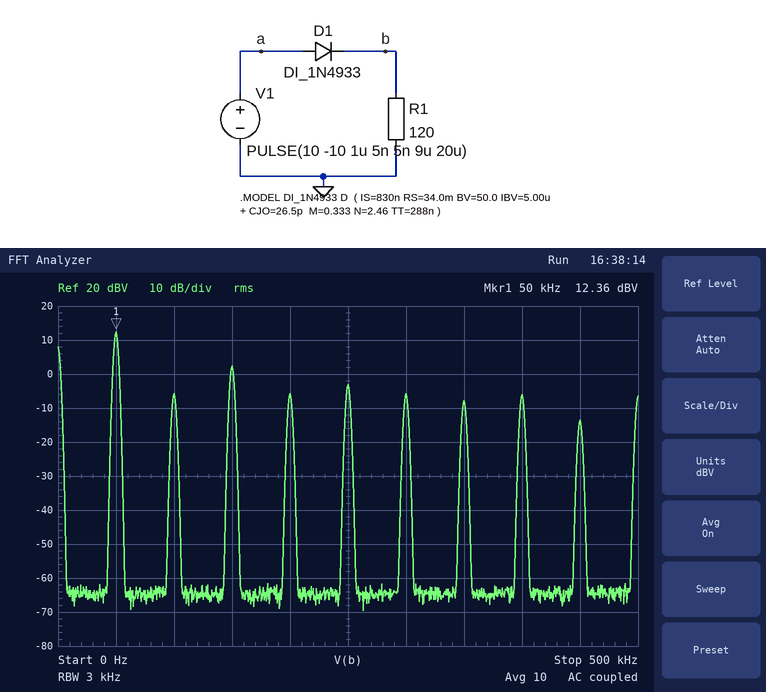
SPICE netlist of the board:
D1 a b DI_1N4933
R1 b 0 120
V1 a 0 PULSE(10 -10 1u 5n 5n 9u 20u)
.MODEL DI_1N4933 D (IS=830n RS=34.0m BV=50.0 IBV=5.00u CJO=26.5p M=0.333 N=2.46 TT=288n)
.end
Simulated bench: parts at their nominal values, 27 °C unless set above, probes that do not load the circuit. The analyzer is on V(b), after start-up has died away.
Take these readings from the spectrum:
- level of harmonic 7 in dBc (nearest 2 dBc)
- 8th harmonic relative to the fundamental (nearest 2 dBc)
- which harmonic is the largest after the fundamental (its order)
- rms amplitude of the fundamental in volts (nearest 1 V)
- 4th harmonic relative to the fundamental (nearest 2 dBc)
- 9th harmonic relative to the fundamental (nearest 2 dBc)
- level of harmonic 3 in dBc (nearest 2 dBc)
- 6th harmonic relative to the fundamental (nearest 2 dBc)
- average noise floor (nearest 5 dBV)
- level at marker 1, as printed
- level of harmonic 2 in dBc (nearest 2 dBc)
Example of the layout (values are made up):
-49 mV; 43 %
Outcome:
-20 dBc; -18 dBc; 3; 4 V; -18 dBc; -26 dBc; -10 dBc; -18 dBc; -65 dBV; 12.36 dBV; -18 dBc
